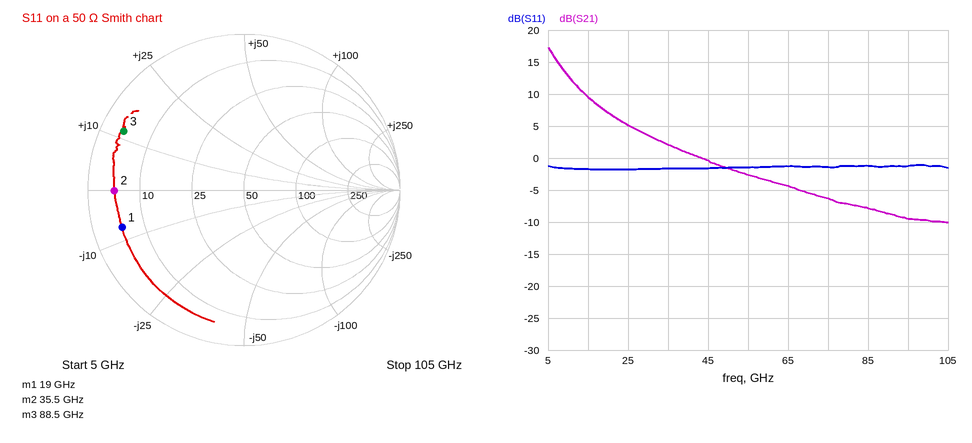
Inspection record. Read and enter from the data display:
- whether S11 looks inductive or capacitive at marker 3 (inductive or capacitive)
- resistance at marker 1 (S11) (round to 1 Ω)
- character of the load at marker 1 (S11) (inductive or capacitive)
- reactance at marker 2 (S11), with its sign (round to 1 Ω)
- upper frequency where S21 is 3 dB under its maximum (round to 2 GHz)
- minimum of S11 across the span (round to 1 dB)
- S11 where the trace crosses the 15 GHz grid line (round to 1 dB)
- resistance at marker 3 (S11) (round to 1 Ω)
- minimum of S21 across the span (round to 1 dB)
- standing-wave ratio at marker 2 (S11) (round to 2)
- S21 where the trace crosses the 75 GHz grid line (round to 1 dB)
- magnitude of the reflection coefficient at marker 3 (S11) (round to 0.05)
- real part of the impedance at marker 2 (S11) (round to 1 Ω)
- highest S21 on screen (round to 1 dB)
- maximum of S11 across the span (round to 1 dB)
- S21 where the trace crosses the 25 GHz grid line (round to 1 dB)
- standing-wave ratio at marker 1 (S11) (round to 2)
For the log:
inductive
5 Ω
capacitive
0 Ω
8 GHz
-2 dB
-2 dB
4 Ω
-10 dB
10
-6 dB
0.85
5 Ω
17 dB
-1 dB
5 dB
10
